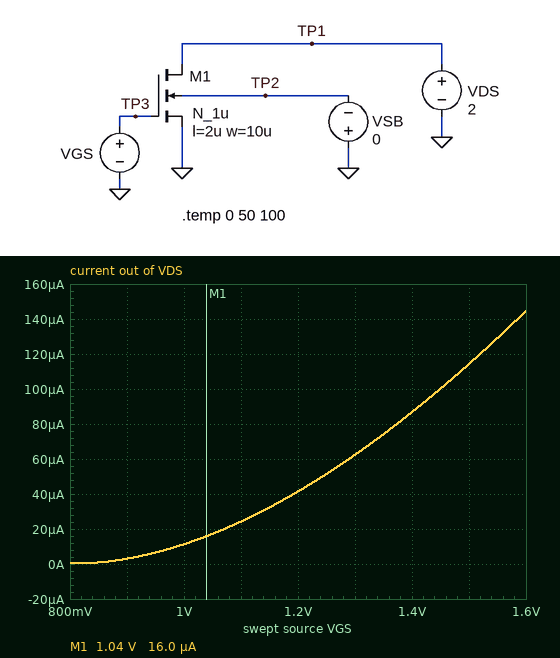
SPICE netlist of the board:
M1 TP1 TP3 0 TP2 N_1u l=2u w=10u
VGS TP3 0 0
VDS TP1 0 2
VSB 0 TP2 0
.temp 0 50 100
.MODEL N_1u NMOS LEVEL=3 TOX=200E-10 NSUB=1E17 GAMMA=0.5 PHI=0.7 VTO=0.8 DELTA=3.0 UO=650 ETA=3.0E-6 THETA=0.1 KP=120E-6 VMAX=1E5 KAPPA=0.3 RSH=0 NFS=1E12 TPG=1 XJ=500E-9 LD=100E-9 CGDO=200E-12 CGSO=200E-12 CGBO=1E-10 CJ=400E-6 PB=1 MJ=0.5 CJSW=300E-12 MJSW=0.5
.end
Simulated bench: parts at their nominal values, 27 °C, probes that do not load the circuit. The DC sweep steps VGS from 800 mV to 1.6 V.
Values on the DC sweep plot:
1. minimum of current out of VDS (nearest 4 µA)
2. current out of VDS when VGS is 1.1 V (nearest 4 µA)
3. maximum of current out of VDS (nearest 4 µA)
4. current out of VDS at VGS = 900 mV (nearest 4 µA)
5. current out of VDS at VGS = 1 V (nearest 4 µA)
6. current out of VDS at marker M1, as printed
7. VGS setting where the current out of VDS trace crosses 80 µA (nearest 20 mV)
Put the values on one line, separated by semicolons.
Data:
0 A; 24 µA; 144 µA; 4 µA; 12 µA; 16.0 µA; 1.38 V
